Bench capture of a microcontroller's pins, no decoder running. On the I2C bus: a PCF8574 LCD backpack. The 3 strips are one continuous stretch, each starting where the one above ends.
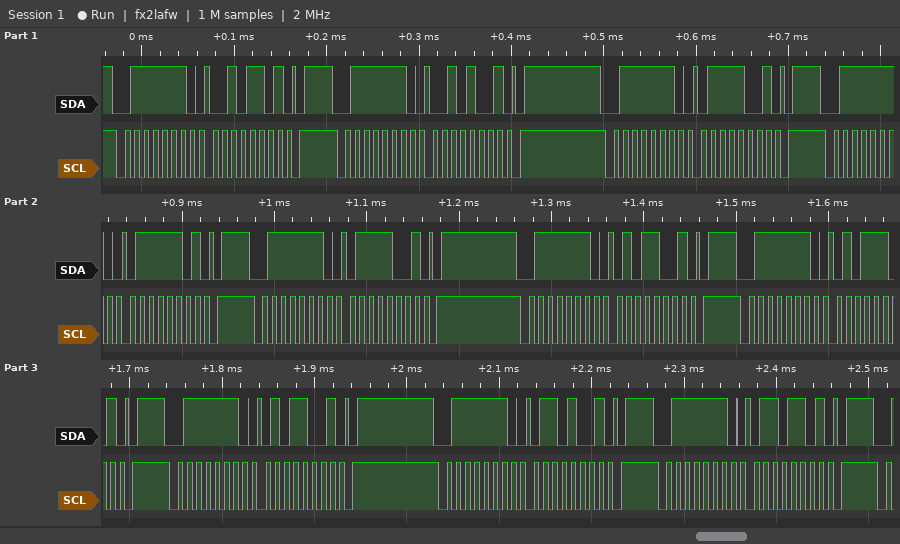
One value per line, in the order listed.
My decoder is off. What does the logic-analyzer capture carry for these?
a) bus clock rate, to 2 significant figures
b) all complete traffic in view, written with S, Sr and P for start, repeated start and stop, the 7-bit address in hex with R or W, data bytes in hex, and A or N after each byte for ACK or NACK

100 kHz
S 3FW A 2D A P S 3FW A 29 A P S 3FW A 79 A P S 3FW A 7D A P S 3FW A 79 A P S 3FW A 59 A P S 3FW A 5D A P S 3FW A 59 A P S 3FW A 69 A P S 3FW A 6D A P
